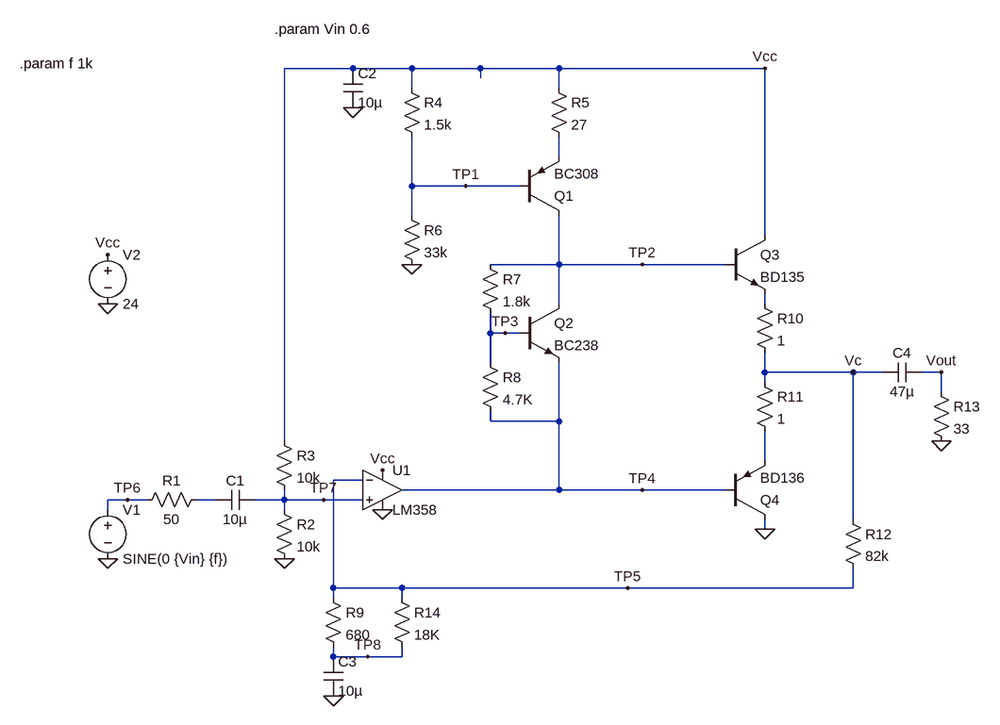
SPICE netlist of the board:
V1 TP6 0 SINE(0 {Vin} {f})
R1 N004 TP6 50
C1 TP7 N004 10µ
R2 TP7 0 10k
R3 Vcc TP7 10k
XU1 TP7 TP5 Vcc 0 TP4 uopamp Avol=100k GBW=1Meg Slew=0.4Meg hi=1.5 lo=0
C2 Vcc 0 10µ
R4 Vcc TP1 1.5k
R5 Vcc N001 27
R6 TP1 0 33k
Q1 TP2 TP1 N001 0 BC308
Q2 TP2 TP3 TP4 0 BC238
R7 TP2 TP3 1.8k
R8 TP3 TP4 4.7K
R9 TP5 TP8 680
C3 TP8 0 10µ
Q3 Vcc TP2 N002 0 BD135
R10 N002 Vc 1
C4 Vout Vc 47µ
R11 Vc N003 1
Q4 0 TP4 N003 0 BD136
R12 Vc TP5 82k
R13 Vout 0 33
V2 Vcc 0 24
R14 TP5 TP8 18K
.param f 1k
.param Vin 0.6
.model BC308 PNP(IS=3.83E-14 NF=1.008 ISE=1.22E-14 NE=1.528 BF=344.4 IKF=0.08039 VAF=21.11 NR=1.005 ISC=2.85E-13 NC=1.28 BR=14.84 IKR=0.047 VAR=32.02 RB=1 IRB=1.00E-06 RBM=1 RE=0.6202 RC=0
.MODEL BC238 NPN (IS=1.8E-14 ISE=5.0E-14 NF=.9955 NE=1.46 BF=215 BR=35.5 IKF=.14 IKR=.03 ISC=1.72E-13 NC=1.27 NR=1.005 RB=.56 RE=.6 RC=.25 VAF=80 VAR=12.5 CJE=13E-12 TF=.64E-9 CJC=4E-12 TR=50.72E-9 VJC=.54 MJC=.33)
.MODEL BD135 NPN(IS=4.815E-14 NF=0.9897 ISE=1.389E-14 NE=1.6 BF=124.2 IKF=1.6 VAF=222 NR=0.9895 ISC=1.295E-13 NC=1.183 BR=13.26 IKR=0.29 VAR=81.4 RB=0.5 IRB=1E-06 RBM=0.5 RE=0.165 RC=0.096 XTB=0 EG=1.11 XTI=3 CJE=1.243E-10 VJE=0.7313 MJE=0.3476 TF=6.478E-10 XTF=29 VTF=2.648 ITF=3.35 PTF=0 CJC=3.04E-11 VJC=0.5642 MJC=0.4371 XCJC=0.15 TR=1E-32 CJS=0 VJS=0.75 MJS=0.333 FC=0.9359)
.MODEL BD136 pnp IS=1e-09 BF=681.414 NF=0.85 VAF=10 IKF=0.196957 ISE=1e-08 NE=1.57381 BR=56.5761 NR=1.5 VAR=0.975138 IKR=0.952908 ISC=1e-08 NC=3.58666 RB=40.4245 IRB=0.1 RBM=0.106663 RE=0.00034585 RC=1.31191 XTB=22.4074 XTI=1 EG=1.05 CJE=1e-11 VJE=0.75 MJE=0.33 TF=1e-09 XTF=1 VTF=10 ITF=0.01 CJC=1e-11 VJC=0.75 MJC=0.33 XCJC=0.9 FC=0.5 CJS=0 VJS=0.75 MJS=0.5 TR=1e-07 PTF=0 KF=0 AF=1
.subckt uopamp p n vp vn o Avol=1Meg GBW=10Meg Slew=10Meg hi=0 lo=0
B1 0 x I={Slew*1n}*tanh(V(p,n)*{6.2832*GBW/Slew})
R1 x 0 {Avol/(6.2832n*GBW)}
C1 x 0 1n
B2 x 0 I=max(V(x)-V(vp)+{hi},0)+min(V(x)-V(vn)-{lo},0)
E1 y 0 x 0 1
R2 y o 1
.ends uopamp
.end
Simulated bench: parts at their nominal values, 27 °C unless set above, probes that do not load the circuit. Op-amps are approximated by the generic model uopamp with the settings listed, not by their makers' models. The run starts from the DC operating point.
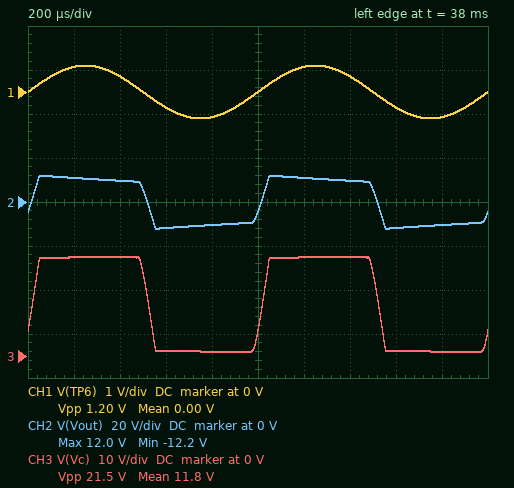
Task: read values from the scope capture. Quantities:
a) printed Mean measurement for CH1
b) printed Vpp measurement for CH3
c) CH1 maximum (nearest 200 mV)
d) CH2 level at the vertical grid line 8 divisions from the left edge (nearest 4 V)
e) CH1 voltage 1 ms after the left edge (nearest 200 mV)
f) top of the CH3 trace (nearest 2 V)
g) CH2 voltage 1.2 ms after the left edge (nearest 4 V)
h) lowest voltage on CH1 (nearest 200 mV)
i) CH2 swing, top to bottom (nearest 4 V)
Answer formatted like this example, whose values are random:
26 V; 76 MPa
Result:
0.00 V; 21.5 V; 600 mV; -12 V; 0 V; 22 V; 12 V; -600 mV; 24 V
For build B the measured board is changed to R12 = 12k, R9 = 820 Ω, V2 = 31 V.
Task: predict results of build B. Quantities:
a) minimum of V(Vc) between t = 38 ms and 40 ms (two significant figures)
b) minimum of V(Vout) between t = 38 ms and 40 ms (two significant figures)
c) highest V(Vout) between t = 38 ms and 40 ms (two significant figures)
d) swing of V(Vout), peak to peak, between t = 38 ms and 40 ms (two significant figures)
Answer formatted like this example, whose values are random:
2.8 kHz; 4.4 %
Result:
5.8 V; -9.6 V; 9.6 V; 19 V
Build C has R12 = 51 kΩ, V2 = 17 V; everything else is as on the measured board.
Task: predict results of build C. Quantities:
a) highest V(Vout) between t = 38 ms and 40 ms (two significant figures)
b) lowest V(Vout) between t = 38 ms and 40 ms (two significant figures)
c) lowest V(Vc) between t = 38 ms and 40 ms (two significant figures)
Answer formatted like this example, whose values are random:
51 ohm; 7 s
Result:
8.1 V; -8.4 V; 750 mV
